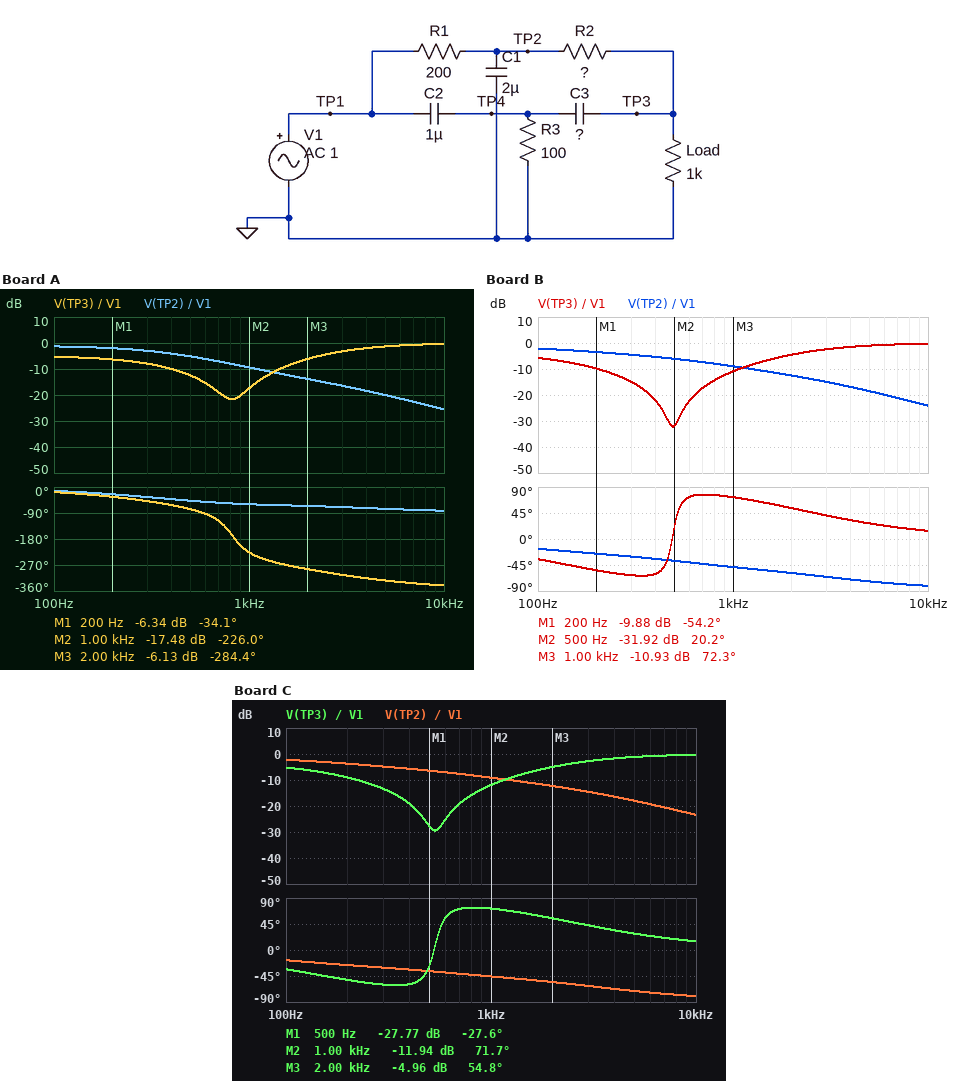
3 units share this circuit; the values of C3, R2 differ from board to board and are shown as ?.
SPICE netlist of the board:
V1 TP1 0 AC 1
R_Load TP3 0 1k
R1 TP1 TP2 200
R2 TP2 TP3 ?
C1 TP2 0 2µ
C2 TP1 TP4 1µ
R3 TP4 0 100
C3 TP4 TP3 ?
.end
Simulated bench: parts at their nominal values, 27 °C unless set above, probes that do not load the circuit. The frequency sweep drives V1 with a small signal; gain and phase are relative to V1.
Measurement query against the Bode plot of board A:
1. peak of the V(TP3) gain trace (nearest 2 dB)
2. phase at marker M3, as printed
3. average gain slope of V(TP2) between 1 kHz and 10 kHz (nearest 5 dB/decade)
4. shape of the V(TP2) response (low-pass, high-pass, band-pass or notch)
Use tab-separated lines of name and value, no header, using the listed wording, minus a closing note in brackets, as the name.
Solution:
peak of the V(TP3) gain trace	0 dB
phase at marker M3, as printed	-284.4 deg
average gain slope of V(TP2) between 1 kHz and 10 kHz	-15 dB/decade
shape of the V(TP2) response	low-pass
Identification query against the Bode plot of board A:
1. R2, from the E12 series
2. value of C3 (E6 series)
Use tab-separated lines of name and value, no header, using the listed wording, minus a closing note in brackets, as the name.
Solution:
R2, from the E12 series	560 Ω
value of C3	330 nF
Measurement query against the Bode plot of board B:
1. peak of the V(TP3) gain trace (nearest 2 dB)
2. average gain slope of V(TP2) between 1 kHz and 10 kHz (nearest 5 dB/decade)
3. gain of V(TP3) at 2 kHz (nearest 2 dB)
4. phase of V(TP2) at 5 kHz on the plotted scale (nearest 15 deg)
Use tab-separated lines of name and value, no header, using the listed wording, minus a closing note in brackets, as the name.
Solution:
peak of the V(TP3) gain trace	0 dB
average gain slope of V(TP2) between 1 kHz and 10 kHz	-15 dB/decade
gain of V(TP3) at 2 kHz	-4 dB
phase of V(TP2) at 5 kHz on the plotted scale	-75 deg
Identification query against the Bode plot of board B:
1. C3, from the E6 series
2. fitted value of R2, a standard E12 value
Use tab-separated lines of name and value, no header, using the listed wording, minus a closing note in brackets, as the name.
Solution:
C3, from the E6 series	2.2 µF
fitted value of R2, a standard E12 value	330 Ω
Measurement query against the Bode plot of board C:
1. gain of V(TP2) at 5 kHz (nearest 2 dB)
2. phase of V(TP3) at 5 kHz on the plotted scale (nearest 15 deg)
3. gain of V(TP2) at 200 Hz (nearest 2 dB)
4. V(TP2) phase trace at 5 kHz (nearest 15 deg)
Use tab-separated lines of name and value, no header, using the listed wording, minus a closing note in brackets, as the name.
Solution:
gain of V(TP2) at 5 kHz	-18 dB
phase of V(TP3) at 5 kHz on the plotted scale	30 deg
gain of V(TP2) at 200 Hz	-4 dB
V(TP2) phase trace at 5 kHz	-75 deg
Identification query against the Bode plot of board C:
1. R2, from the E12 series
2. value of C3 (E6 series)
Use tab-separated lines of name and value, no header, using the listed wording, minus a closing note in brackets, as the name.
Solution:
R2, from the E12 series	270 Ω
value of C3	2.2 µF
